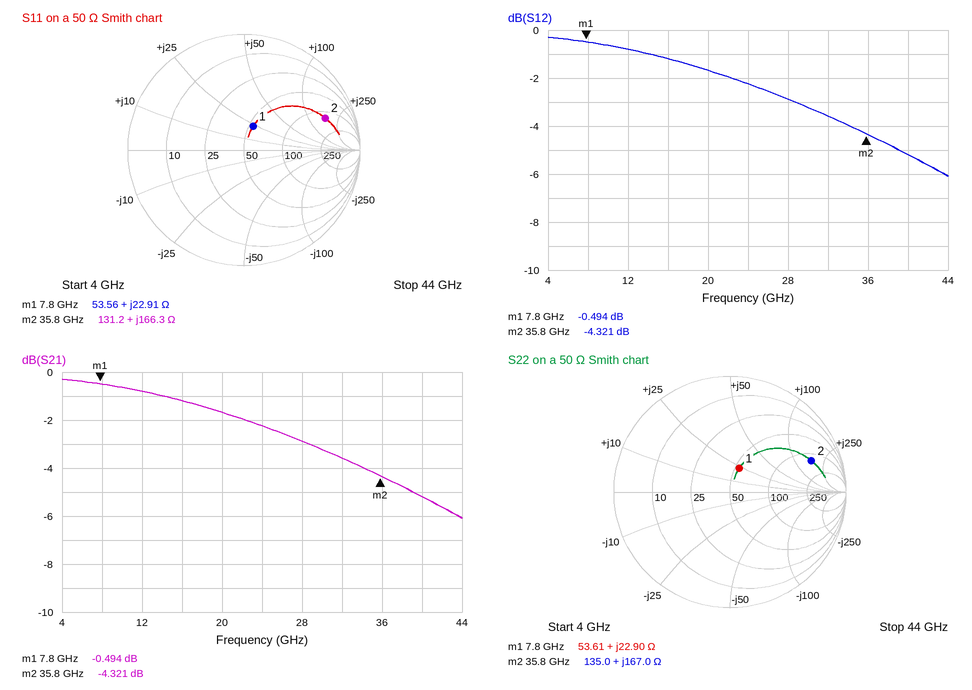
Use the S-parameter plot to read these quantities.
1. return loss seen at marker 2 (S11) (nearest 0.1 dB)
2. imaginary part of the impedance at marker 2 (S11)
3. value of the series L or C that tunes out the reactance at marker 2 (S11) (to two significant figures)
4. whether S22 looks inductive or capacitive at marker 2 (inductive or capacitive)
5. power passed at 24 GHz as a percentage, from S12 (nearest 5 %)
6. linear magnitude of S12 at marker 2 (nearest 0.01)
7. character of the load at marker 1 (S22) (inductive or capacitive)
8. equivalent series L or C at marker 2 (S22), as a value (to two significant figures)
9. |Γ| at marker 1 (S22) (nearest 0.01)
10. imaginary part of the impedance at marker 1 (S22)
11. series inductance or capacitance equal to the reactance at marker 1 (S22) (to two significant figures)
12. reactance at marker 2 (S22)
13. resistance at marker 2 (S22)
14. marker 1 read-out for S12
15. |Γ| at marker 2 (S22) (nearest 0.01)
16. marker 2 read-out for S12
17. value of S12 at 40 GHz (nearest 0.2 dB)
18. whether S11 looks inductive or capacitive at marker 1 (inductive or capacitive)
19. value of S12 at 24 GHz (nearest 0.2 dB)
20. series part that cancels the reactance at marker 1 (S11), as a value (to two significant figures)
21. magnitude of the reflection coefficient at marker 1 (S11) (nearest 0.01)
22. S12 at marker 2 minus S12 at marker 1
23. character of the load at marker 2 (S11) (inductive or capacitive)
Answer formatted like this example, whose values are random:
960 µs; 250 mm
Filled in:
2.5 dB; +166.3 Ω; 27 fF; inductive; 60 %; 0.61; inductive; 740 pH; 0.22; +22.90 Ω; 470 pH; +167.0 Ω; 135.0 Ω; -0.494 dB; 0.75; -4.321 dB; -5.2 dB; inductive; -2.2 dB; 890 fF; 0.22; -3.827 dB; inductive
